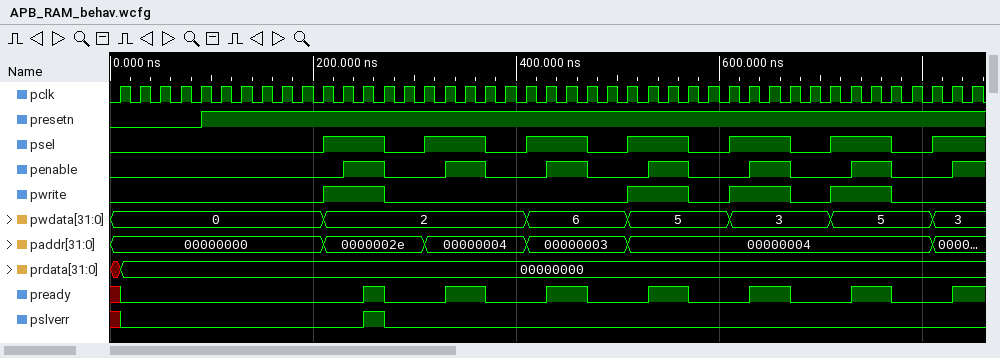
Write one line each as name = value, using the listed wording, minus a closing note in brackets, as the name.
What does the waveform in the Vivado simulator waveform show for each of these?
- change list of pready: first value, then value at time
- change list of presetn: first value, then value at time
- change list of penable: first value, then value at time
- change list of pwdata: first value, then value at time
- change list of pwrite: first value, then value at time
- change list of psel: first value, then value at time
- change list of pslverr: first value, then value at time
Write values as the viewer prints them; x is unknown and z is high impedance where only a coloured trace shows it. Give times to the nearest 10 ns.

change list of pready: first value, then value at time = x, 0 at 10 ns, 1 at 250 ns, 0 at 270 ns, 1 at 330 ns, 0 at 370 ns, 1 at 430 ns, 0 at 470 ns, 1 at 530 ns, 0 at 570 ns, 1 at 630 ns, 0 at 670 ns, 1 at 730 ns, 0 at 770 ns, 1 at 830 ns
change list of presetn: first value, then value at time = 0, 1 at 90 ns
change list of penable: first value, then value at time = 0, 1 at 230 ns, 0 at 270 ns, 1 at 330 ns, 0 at 370 ns, 1 at 430 ns, 0 at 470 ns, 1 at 530 ns, 0 at 570 ns, 1 at 630 ns, 0 at 670 ns, 1 at 730 ns, 0 at 770 ns, 1 at 830 ns
change list of pwdata: first value, then value at time = 0, 2 at 210 ns, 6 at 410 ns, 5 at 510 ns, 3 at 610 ns, 5 at 710 ns, 3 at 810 ns
change list of pwrite: first value, then value at time = 0, 1 at 210 ns, 0 at 270 ns, 1 at 510 ns, 0 at 570 ns, 1 at 610 ns, 0 at 670 ns, 1 at 710 ns, 0 at 770 ns
change list of psel: first value, then value at time = 0, 1 at 210 ns, 0 at 270 ns, 1 at 310 ns, 0 at 370 ns, 1 at 410 ns, 0 at 470 ns, 1 at 510 ns, 0 at 570 ns, 1 at 610 ns, 0 at 670 ns, 1 at 710 ns, 0 at 770 ns, 1 at 810 ns
change list of pslverr: first value, then value at time = x, 0 at 10 ns, 1 at 250 ns, 0 at 270 ns
